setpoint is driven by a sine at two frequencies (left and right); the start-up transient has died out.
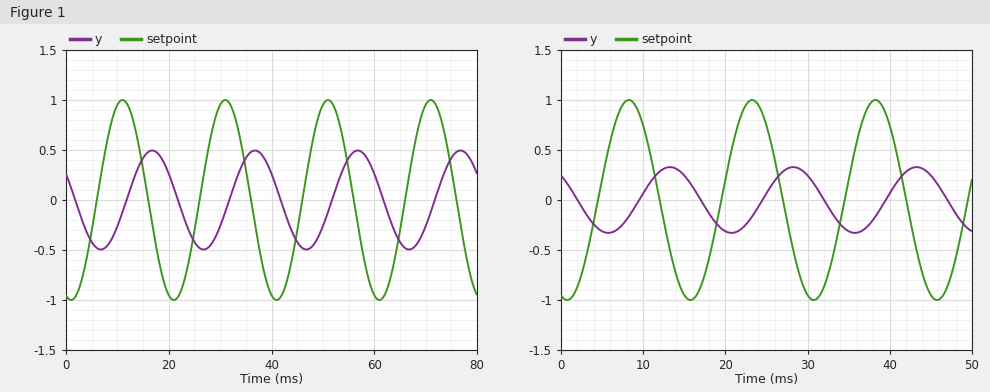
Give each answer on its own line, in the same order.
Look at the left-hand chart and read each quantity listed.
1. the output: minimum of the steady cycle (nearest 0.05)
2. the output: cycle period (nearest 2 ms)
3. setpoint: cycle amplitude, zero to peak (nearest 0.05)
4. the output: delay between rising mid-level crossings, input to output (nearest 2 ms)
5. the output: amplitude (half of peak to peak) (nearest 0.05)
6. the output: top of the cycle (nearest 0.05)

-0.50
20 ms
1.00
6 ms
0.50
0.50
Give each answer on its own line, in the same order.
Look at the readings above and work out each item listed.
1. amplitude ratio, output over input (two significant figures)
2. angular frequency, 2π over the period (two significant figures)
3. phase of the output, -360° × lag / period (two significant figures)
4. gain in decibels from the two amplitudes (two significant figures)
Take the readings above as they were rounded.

0.50
0.31 rad/ms
-110°
-6.0 dB
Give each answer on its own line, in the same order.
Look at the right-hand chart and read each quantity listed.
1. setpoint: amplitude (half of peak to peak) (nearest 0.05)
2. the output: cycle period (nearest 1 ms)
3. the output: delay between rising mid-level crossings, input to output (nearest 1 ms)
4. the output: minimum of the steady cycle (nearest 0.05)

1.00
15 ms
5 ms
-0.35
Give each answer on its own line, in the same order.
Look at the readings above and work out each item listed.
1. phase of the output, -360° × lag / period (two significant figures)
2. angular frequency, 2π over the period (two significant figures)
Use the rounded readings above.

-120°
0.42 rad/ms
